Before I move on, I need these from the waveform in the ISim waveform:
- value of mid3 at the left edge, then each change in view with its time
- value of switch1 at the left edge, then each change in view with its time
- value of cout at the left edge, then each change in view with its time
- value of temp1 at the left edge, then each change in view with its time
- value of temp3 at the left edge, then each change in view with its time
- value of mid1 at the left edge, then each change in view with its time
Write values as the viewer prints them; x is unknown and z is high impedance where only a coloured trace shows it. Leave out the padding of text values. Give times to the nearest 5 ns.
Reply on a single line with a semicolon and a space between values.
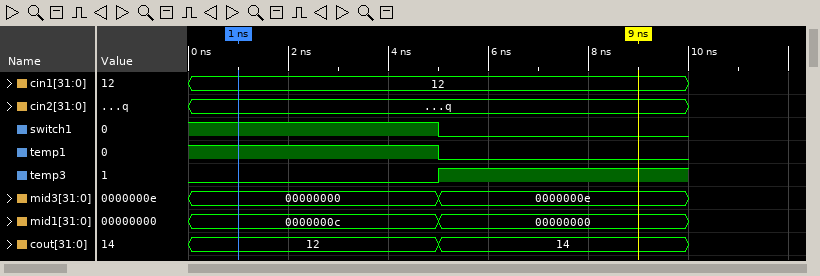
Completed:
00000000, 0000000e at 5 ns; 1, 0 at 5 ns; 12, 14 at 5 ns; 1, 0 at 5 ns; 0, 1 at 5 ns; 0000000c, 00000000 at 5 ns
